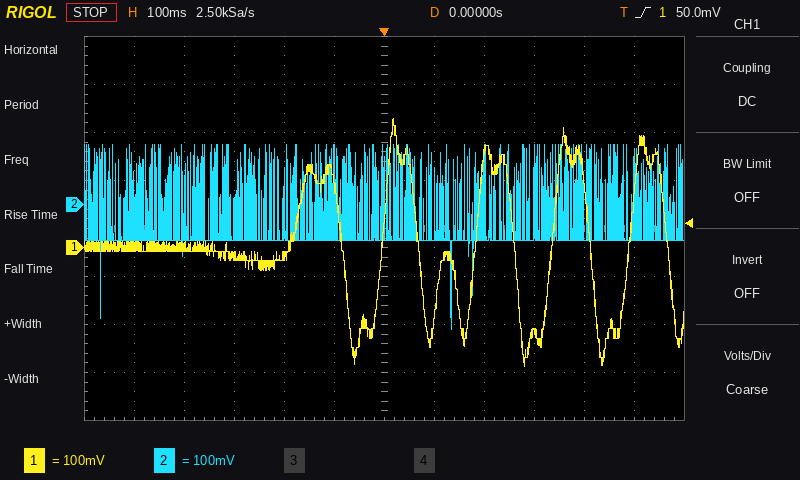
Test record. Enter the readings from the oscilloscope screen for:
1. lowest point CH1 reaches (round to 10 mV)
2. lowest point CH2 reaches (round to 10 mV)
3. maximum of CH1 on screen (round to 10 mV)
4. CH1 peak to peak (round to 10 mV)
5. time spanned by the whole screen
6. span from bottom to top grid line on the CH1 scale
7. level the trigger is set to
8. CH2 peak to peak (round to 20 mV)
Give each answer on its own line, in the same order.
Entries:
-250 mV
-260 mV
270 mV
520 mV
1.2 s
800 mV
50.0 mV
380 mV
